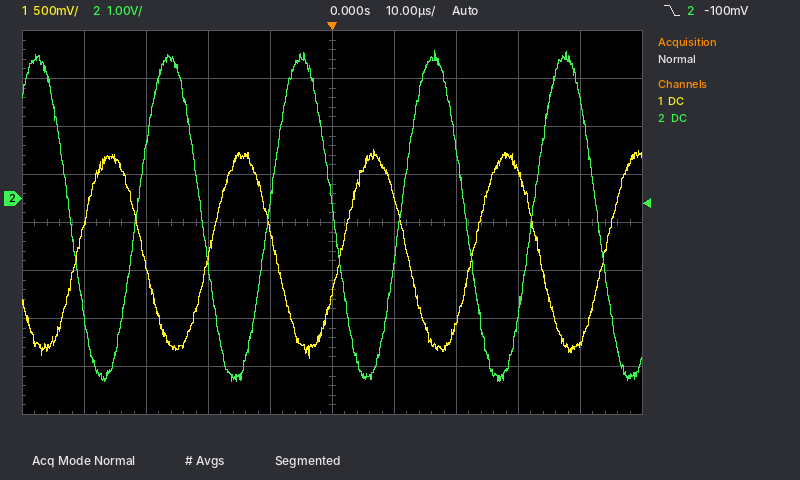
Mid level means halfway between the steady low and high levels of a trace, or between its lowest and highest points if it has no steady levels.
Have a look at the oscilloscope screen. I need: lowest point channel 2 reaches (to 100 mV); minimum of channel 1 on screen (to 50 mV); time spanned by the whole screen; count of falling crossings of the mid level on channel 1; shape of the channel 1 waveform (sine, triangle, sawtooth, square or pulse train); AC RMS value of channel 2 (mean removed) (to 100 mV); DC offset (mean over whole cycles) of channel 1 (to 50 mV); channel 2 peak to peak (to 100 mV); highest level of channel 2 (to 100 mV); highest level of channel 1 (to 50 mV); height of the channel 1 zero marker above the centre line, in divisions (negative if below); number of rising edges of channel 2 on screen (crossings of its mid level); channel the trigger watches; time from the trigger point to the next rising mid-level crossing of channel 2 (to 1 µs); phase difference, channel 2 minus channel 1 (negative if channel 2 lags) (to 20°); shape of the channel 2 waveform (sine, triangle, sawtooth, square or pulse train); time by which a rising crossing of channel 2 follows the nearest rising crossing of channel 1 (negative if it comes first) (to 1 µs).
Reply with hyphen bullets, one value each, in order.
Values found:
- -3.8 V
- -1.65 V
- 100 µs
- 4
- sine
- 2.4 V
- -550 mV
- 6.9 V
- 3.1 V
- 500 mV
- +0.5 div
- 4
- channel 2
- 11 µs
- -160°
- sine
- +10 µs
